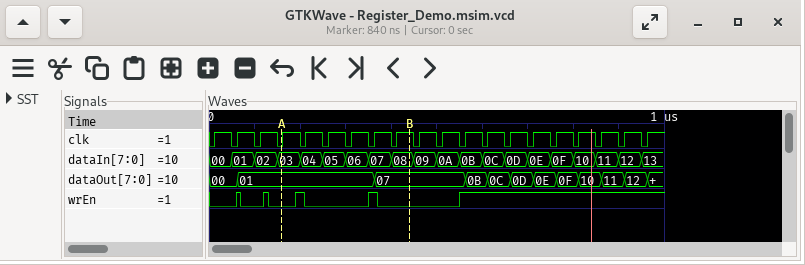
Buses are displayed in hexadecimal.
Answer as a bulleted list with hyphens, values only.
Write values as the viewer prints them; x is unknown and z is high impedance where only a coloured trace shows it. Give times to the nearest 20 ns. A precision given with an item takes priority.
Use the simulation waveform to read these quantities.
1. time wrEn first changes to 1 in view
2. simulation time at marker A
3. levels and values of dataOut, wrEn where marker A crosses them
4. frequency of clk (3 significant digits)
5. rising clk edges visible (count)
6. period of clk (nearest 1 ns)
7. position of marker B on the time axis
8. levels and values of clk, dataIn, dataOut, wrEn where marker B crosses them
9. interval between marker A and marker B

- 60 ns
- 160 ns
- dataOut=01, wrEn=0
- 20.0 MHz
- 20
- 50 ns
- 440 ns
- clk=1, dataIn=08, dataOut=07, wrEn=0
- 280 ns
